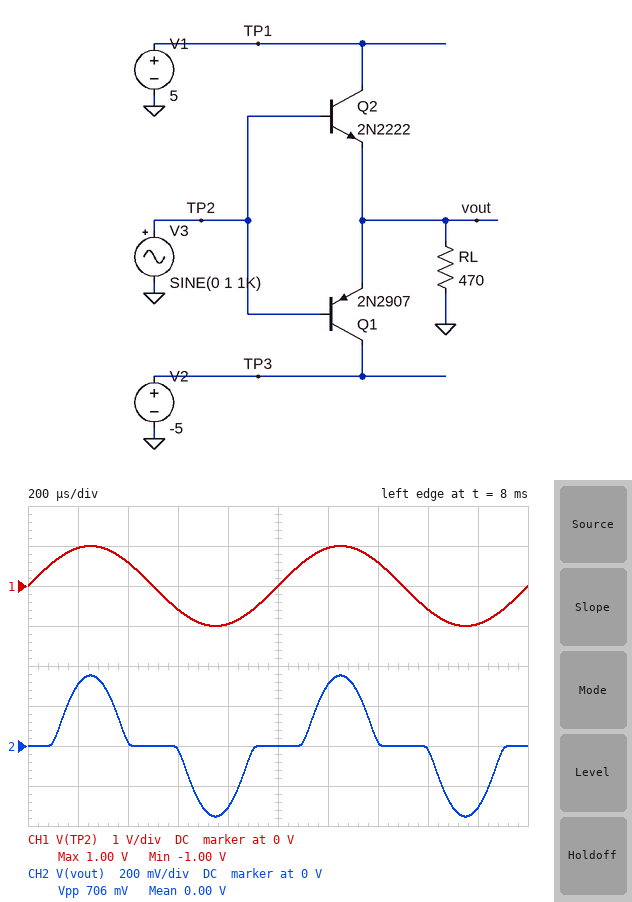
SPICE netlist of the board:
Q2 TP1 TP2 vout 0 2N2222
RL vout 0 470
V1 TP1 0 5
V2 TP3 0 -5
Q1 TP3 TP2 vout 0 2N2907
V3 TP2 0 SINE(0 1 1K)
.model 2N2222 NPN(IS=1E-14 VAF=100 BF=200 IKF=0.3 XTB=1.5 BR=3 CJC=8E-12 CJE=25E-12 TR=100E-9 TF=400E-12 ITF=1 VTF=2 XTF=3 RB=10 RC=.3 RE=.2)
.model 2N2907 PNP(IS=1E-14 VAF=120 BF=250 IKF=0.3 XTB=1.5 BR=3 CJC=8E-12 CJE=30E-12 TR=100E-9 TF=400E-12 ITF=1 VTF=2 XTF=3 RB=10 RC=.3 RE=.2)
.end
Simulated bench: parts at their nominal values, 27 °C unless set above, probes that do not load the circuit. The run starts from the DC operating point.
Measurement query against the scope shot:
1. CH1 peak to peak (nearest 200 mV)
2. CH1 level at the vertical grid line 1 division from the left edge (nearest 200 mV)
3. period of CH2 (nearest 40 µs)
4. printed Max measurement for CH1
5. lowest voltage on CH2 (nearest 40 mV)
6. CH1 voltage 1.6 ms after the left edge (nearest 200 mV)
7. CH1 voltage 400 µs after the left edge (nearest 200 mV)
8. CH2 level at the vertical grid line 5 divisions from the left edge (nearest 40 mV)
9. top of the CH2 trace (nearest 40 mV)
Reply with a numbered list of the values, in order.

1. 2.0 V
2. 1.0 V
3. 1.00 ms
4. 1.00 V
5. -360 mV
6. -600 mV
7. 600 mV
8. 0 V
9. 360 mV
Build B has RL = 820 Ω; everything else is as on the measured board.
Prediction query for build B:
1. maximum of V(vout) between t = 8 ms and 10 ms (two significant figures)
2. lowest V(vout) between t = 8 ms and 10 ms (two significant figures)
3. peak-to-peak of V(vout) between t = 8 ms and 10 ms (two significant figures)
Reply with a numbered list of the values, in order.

1. 370 mV
2. -370 mV
3. 730 mV
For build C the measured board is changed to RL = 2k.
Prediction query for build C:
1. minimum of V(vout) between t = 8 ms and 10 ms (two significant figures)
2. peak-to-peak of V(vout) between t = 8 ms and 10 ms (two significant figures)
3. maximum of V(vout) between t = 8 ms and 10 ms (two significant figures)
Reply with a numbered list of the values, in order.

1. -390 mV
2. 780 mV
3. 390 mV
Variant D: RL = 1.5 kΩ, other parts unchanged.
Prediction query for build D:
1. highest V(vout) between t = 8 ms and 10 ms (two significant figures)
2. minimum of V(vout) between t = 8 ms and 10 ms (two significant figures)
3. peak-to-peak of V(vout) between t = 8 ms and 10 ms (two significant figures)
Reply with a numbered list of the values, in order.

1. 380 mV
2. -380 mV
3. 760 mV
